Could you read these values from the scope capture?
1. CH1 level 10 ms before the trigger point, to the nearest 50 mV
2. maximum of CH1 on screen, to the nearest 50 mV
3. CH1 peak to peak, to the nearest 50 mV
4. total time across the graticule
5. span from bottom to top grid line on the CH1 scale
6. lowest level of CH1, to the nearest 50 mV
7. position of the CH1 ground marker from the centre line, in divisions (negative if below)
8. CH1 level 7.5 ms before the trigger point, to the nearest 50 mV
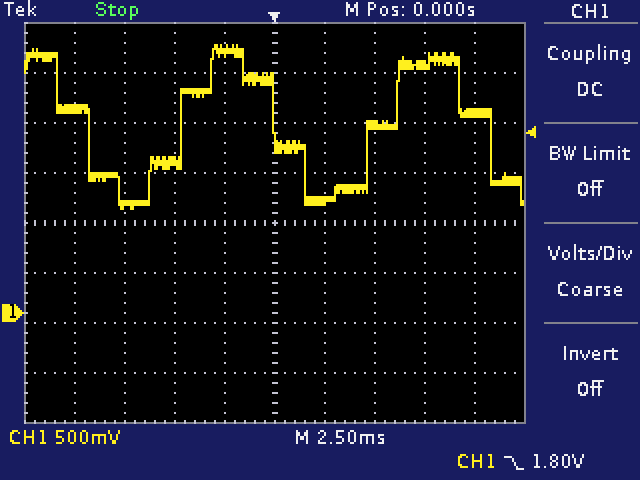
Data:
2.05 V
2.70 V
1.65 V
25 ms
4 V
1.05 V
-1.8 div
1.10 V
